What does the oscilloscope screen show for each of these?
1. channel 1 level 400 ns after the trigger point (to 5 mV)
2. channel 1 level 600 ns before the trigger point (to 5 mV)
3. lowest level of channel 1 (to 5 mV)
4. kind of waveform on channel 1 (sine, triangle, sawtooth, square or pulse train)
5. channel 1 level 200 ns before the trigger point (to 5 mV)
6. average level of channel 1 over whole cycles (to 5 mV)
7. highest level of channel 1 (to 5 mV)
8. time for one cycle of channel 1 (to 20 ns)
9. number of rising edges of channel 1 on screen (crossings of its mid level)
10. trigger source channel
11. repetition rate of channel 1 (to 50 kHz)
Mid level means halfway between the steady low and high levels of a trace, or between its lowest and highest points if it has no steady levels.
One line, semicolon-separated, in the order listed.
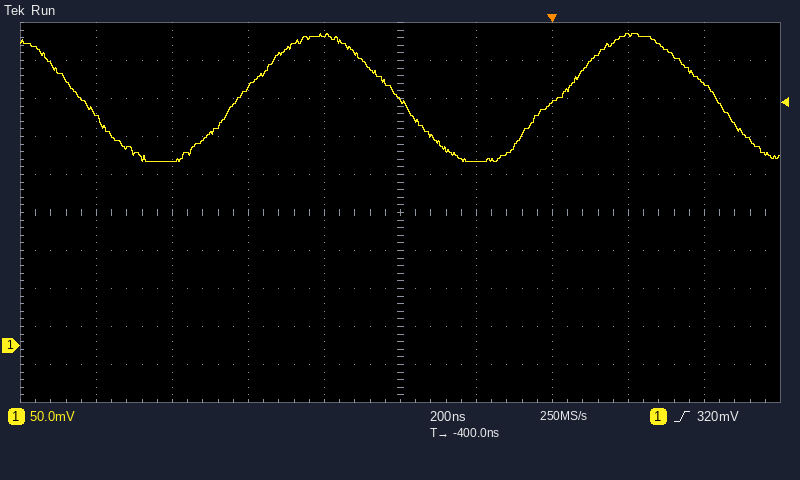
345 mV; 410 mV; 240 mV; sine; 240 mV; 325 mV; 410 mV; 840 ns; 2; channel 1; 1.20 MHz
